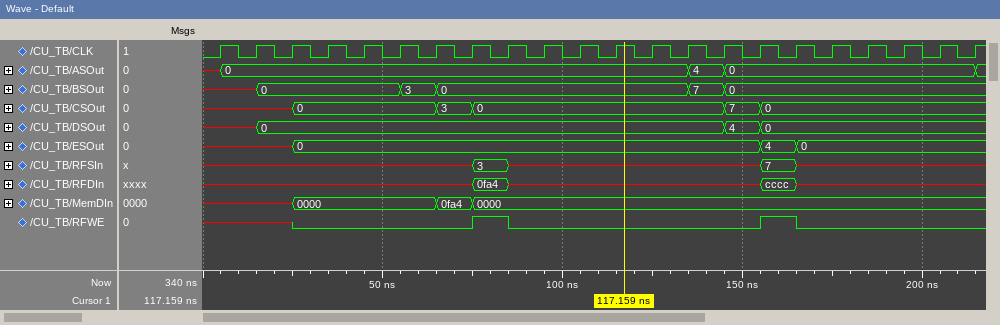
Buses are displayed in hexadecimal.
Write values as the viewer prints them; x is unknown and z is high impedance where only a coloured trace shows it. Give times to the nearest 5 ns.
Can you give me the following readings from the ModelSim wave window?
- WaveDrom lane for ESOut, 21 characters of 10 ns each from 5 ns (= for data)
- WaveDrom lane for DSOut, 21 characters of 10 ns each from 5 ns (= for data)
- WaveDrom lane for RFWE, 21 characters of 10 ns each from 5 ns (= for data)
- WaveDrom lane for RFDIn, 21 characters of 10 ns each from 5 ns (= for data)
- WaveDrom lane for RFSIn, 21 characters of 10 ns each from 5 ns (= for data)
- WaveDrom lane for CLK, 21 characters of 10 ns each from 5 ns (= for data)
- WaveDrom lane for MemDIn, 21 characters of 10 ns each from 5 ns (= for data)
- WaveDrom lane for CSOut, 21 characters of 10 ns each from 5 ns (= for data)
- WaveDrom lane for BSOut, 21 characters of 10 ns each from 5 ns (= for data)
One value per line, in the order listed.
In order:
{name: 'ESOut', wave: 'x.=............==....', data: '0 4 0'}
{name: 'DSOut', wave: 'x=............==.....', data: '0 4 0'}
{name: 'RFWE', wave: 'x.0....10......10....'}
{name: 'RFDIn', wave: 'x......=x......=x....', data: '0fa4 cccc'}
{name: 'RFSIn', wave: 'x......=x......=x....', data: '3 7'}
{name: 'CLK', wave: 'p....................'}
{name: 'MemDIn', wave: 'x.=...==.............', data: '0000 0fa4 0000'}
{name: 'CSOut', wave: 'x.=...==......==.....', data: '0 3 0 7 0'}
{name: 'BSOut', wave: 'x=...==......==......', data: '0 3 0 7 0'}
